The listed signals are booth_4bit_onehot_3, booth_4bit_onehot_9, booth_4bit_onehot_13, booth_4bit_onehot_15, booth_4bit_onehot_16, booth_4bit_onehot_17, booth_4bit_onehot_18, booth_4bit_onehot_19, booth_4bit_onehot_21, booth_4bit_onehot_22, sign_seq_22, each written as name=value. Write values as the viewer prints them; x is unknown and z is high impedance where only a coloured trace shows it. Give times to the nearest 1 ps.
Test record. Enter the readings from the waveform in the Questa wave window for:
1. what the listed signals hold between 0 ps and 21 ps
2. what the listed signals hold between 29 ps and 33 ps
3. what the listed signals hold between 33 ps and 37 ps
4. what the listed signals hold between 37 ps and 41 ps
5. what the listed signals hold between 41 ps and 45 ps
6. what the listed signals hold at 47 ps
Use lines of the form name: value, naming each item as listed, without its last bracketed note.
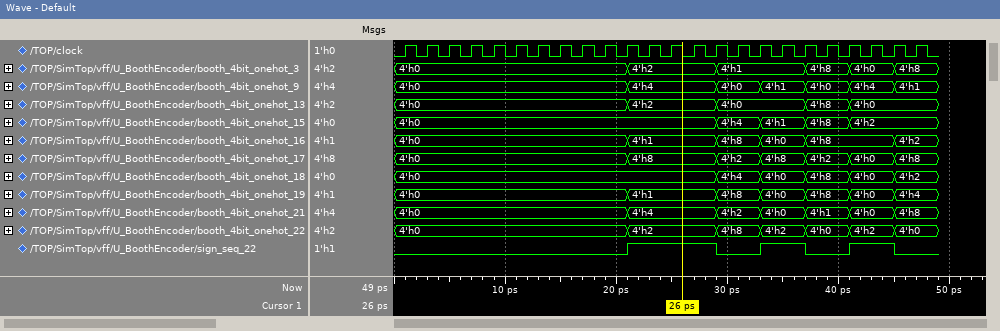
what the listed signals hold between 0 ps and 21 ps: booth_4bit_onehot_3=4'h0, booth_4bit_onehot_9=4'h0, booth_4bit_onehot_13=4'h0, booth_4bit_onehot_15=4'h0, booth_4bit_onehot_16=4'h0, booth_4bit_onehot_17=4'h0, booth_4bit_onehot_18=4'h0, booth_4bit_onehot_19=4'h0, booth_4bit_onehot_21=4'h0, booth_4bit_onehot_22=4'h0, sign_seq_22=0
what the listed signals hold between 29 ps and 33 ps: booth_4bit_onehot_3=4'h1, booth_4bit_onehot_9=4'h0, booth_4bit_onehot_13=4'h0, booth_4bit_onehot_15=4'h4, booth_4bit_onehot_16=4'h8, booth_4bit_onehot_17=4'h2, booth_4bit_onehot_18=4'h4, booth_4bit_onehot_19=4'h8, booth_4bit_onehot_21=4'h2, booth_4bit_onehot_22=4'h8, sign_seq_22=0
what the listed signals hold between 33 ps and 37 ps: booth_4bit_onehot_3=4'h1, booth_4bit_onehot_9=4'h1, booth_4bit_onehot_13=4'h0, booth_4bit_onehot_15=4'h1, booth_4bit_onehot_16=4'h0, booth_4bit_onehot_17=4'h8, booth_4bit_onehot_18=4'h0, booth_4bit_onehot_19=4'h0, booth_4bit_onehot_21=4'h0, booth_4bit_onehot_22=4'h2, sign_seq_22=1
what the listed signals hold between 37 ps and 41 ps: booth_4bit_onehot_3=4'h8, booth_4bit_onehot_9=4'h0, booth_4bit_onehot_13=4'h8, booth_4bit_onehot_15=4'h8, booth_4bit_onehot_16=4'h8, booth_4bit_onehot_17=4'h2, booth_4bit_onehot_18=4'h8, booth_4bit_onehot_19=4'h8, booth_4bit_onehot_21=4'h1, booth_4bit_onehot_22=4'h0, sign_seq_22=0
what the listed signals hold between 41 ps and 45 ps: booth_4bit_onehot_3=4'h0, booth_4bit_onehot_9=4'h4, booth_4bit_onehot_13=4'h0, booth_4bit_onehot_15=4'h2, booth_4bit_onehot_16=4'h8, booth_4bit_onehot_17=4'h0, booth_4bit_onehot_18=4'h0, booth_4bit_onehot_19=4'h0, booth_4bit_onehot_21=4'h0, booth_4bit_onehot_22=4'h2, sign_seq_22=1
what the listed signals hold at 47 ps: booth_4bit_onehot_3=4'h8, booth_4bit_onehot_9=4'h1, booth_4bit_onehot_13=4'h0, booth_4bit_onehot_15=4'h2, booth_4bit_onehot_16=4'h2, booth_4bit_onehot_17=4'h8, booth_4bit_onehot_18=4'h2, booth_4bit_onehot_19=4'h4, booth_4bit_onehot_21=4'h8, booth_4bit_onehot_22=4'h0, sign_seq_22=0
